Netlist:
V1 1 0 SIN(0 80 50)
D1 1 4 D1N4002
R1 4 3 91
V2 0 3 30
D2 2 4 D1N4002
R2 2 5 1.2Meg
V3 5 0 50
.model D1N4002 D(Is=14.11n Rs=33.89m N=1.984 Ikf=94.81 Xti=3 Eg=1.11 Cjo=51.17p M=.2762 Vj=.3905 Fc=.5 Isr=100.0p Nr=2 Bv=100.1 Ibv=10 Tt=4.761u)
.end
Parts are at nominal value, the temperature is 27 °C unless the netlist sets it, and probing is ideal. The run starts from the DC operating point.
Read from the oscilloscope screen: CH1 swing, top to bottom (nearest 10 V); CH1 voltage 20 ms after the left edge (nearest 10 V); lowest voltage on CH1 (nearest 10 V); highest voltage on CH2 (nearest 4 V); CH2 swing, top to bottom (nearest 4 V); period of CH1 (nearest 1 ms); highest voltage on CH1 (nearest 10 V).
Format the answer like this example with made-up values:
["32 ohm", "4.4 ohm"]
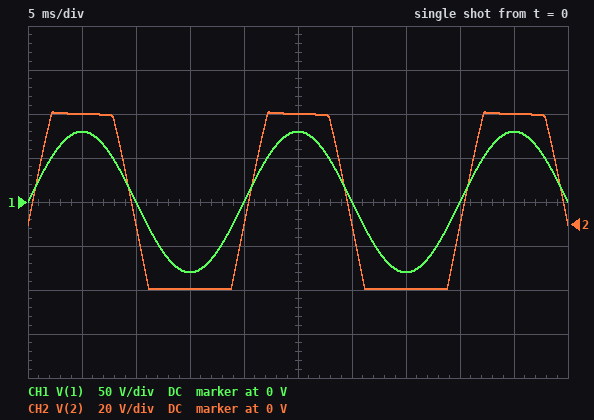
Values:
["160 V", "0 V", "-80 V", "52 V", "80 V", "20 ms", "80 V"]
